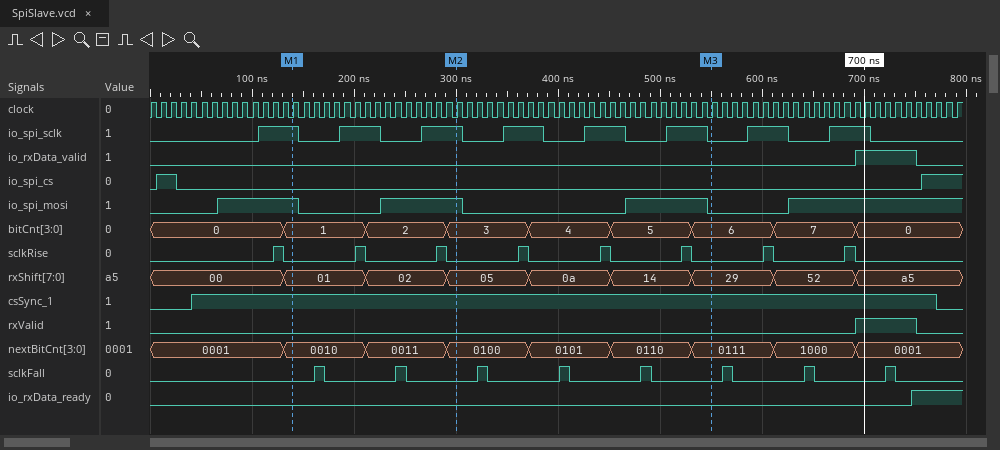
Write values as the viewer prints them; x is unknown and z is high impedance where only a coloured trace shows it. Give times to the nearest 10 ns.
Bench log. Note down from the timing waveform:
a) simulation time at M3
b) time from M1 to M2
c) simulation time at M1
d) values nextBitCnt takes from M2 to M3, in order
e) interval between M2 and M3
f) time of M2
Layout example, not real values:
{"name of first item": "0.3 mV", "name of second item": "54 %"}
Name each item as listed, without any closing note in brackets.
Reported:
{"simulation time at M3": "550 ns", "time from M1 to M2": "160 ns", "simulation time at M1": "140 ns", "values nextBitCnt takes from M2 to M3, in order": "0100, 0101, 0110, 0111", "interval between M2 and M3": "250 ns", "time of M2": "300 ns"}
